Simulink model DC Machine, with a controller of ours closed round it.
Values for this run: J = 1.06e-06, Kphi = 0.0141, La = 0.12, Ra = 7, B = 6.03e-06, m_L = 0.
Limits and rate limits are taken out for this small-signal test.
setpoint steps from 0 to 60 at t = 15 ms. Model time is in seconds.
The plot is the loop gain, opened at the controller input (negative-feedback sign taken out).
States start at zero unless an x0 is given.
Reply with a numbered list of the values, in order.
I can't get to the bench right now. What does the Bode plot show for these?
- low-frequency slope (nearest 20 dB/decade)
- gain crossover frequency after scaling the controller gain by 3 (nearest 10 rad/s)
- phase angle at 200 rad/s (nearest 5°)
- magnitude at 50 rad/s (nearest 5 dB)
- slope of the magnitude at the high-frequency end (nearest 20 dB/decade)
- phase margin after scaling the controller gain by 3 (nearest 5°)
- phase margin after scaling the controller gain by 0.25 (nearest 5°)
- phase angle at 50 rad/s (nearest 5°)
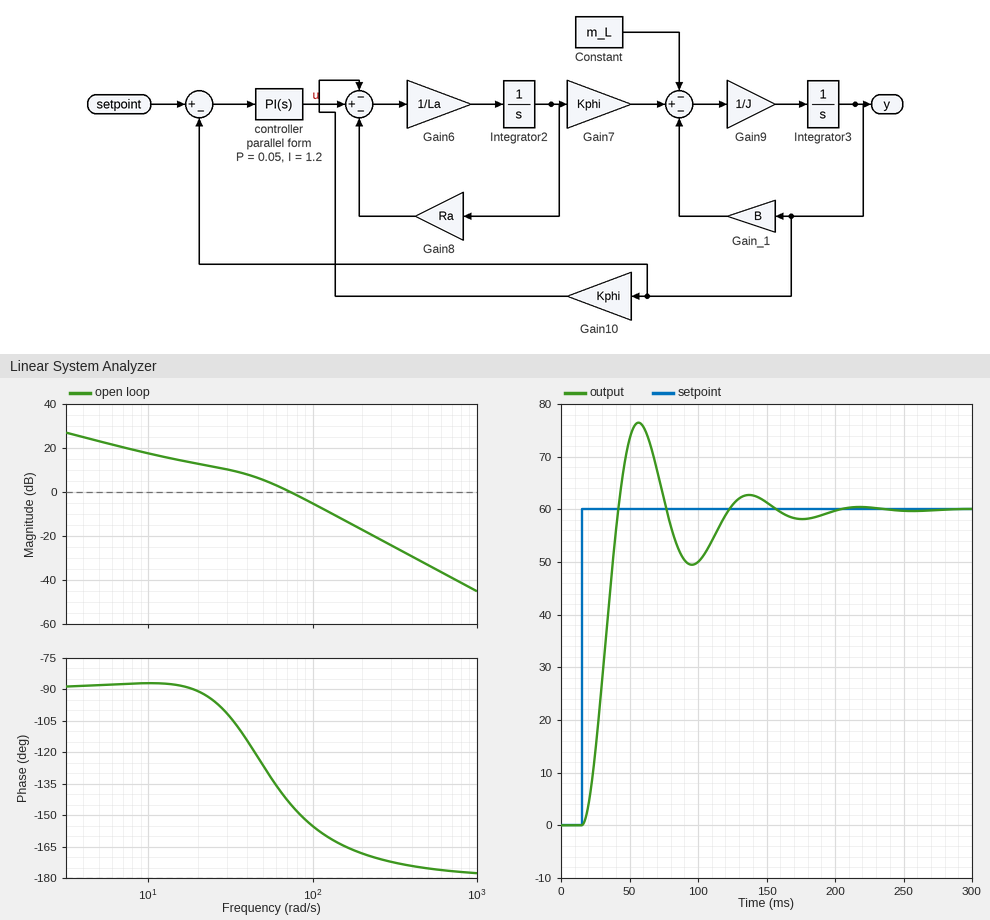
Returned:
1. -20 dB/decade
2. 130 rad/s
3. -170°
4. 5 dB
5. -40 dB/decade
6. 20°
7. 85°
8. -125°
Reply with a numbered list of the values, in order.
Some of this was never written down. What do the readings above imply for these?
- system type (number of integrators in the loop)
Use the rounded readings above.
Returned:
1. 1
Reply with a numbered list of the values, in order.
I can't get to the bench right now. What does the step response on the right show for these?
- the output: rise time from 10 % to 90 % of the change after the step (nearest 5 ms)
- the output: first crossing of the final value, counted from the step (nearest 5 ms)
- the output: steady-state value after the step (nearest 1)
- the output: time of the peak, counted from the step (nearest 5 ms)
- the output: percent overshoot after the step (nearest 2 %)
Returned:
1. 20 ms
2. 25 ms
3. 60
4. 40 ms
5. 28 %
